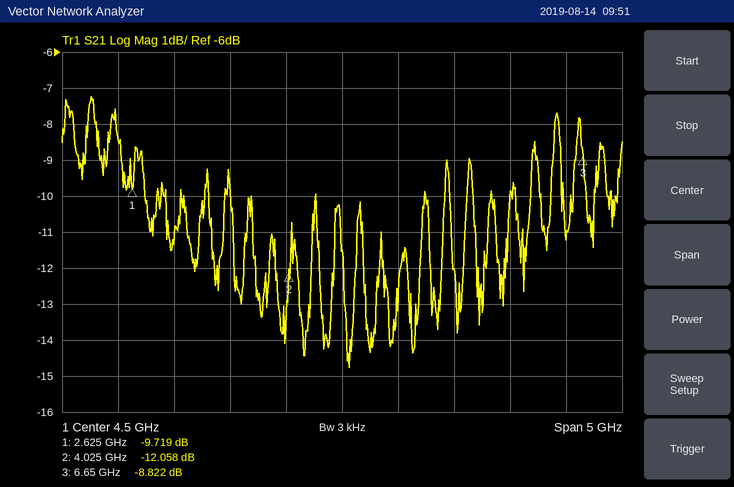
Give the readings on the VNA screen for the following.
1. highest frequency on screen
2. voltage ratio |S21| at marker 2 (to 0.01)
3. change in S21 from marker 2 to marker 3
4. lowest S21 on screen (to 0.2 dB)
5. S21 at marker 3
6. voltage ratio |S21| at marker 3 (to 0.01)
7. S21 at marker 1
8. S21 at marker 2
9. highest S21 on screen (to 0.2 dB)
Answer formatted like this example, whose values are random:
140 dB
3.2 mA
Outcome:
7 GHz
0.25
3.236 dB
-14.8 dB
-8.822 dB
0.36
-9.719 dB
-12.058 dB
-7.2 dB
